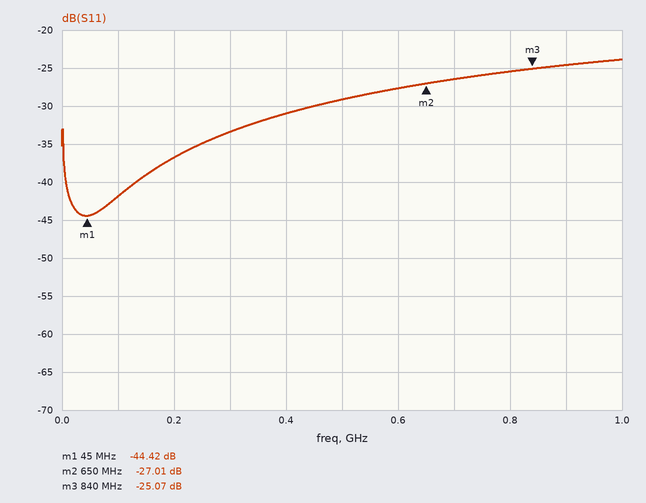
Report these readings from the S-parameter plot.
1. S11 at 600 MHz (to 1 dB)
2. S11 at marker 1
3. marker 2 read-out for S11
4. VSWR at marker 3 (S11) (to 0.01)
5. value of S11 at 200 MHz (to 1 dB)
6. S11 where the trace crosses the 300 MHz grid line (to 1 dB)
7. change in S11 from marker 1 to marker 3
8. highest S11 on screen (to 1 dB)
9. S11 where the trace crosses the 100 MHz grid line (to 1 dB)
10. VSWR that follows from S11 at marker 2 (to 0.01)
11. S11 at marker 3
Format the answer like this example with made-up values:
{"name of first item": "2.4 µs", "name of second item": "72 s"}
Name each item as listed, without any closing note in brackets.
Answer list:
{"S11 at 600 MHz": "-28 dB", "S11 at marker 1": "-44.42 dB", "marker 2 read-out for S11": "-27.01 dB", "VSWR at marker 3 (S11)": "1.12", "value of S11 at 200 MHz": "-37 dB", "S11 where the trace crosses the 300 MHz grid line": "-33 dB", "change in S11 from marker 1 to marker 3": "19.35 dB", "highest S11 on screen": "-24 dB", "S11 where the trace crosses the 100 MHz grid line": "-42 dB", "VSWR that follows from S11 at marker 2": "1.09", "S11 at marker 3": "-25.07 dB"}
